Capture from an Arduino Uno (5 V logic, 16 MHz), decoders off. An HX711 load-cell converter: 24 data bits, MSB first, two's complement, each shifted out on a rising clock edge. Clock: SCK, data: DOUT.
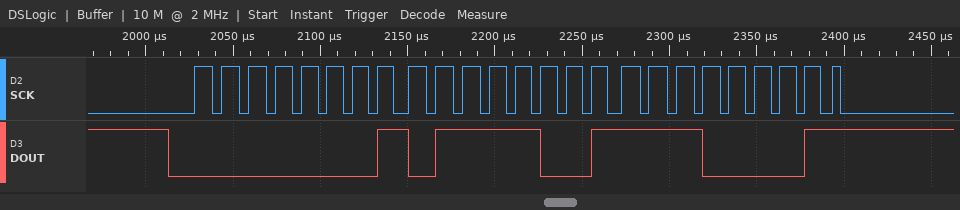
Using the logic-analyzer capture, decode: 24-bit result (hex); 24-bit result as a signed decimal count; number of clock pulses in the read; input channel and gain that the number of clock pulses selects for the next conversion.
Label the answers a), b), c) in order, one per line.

a) 0x0179E1
b) 96737
c) 25
d) channel A, gain 128
